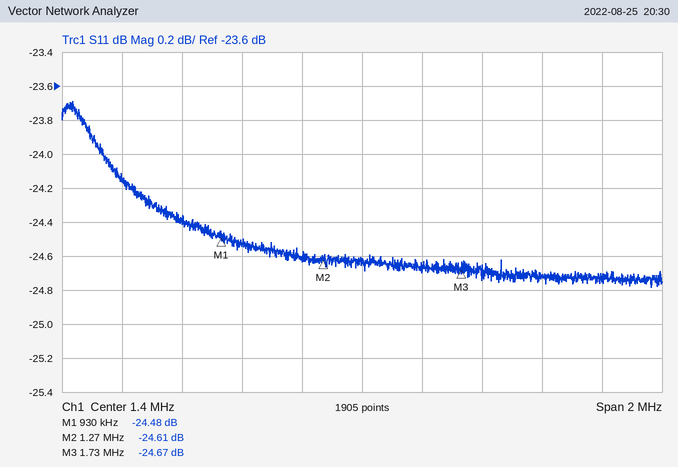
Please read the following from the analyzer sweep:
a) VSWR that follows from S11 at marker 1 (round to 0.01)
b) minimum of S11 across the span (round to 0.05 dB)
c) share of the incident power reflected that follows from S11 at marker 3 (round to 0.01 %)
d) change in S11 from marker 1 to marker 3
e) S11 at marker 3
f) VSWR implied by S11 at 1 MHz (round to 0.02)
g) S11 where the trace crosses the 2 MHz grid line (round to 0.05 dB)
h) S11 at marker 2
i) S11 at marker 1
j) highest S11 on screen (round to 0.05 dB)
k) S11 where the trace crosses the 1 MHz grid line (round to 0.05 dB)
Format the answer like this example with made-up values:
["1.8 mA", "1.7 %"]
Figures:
["1.13", "-24.80 dB", "0.34 %", "-0.19 dB", "-24.67 dB", "1.12", "-24.70 dB", "-24.61 dB", "-24.48 dB", "-23.70 dB", "-24.55 dB"]
